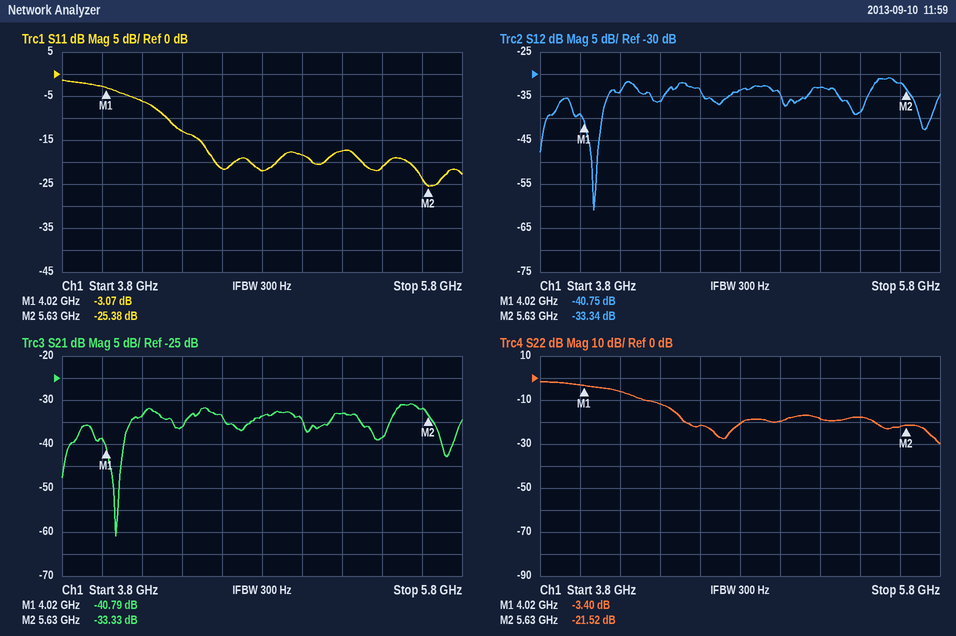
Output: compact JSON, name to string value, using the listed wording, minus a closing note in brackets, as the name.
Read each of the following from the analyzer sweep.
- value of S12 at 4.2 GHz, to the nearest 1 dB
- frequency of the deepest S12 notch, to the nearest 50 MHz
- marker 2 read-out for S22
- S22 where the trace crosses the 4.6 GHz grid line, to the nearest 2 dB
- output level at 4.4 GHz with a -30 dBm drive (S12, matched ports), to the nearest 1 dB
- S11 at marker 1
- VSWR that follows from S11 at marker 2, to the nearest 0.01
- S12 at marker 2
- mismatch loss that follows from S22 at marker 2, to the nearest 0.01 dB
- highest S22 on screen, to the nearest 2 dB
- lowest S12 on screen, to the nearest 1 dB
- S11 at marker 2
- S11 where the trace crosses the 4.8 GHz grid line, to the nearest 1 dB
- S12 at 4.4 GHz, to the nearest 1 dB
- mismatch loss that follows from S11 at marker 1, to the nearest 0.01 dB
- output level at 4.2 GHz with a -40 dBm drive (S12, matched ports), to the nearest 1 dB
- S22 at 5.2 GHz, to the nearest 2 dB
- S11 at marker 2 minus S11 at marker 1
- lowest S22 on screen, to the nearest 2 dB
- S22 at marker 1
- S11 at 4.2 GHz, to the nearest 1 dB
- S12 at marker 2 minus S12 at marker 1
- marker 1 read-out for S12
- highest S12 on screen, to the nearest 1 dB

{"value of S12 at 4.2 GHz, to the nearest 1 dB": "-34 dB", "frequency of the deepest S12 notch, to the nearest 50 MHz": "4.05 GHz", "marker 2 read-out for S22": "-21.52 dB", "S22 where the trace crosses the 4.6 GHz grid line, to the nearest 2 dB": "-22 dB", "output level at 4.4 GHz with a -30 dBm drive (S12, matched ports), to the nearest 1 dB": "-66 dBm", "S11 at marker 1": "-3.07 dB", "VSWR that follows from S11 at marker 2, to the nearest 0.01": "1.11", "S12 at marker 2": "-33.34 dB", "mismatch loss that follows from S22 at marker 2, to the nearest 0.01 dB": "0.03 dB", "highest S22 on screen, to the nearest 2 dB": "-2 dB", "lowest S12 on screen, to the nearest 1 dB": "-61 dB", "S11 at marker 2": "-25.38 dB", "S11 where the trace crosses the 4.8 GHz grid line, to the nearest 1 dB": "-22 dB", "S12 at 4.4 GHz, to the nearest 1 dB": "-36 dB", "mismatch loss that follows from S11 at marker 1, to the nearest 0.01 dB": "2.95 dB", "output level at 4.2 GHz with a -40 dBm drive (S12, matched ports), to the nearest 1 dB": "-74 dBm", "S22 at 5.2 GHz, to the nearest 2 dB": "-18 dB", "S11 at marker 2 minus S11 at marker 1": "-22.31 dB", "lowest S22 on screen, to the nearest 2 dB": "-30 dB", "S22 at marker 1": "-3.40 dB", "S11 at 4.2 GHz, to the nearest 1 dB": "-6 dB", "S12 at marker 2 minus S12 at marker 1": "7.41 dB", "marker 1 read-out for S12": "-40.75 dB", "highest S12 on screen, to the nearest 1 dB": "-31 dB"}
